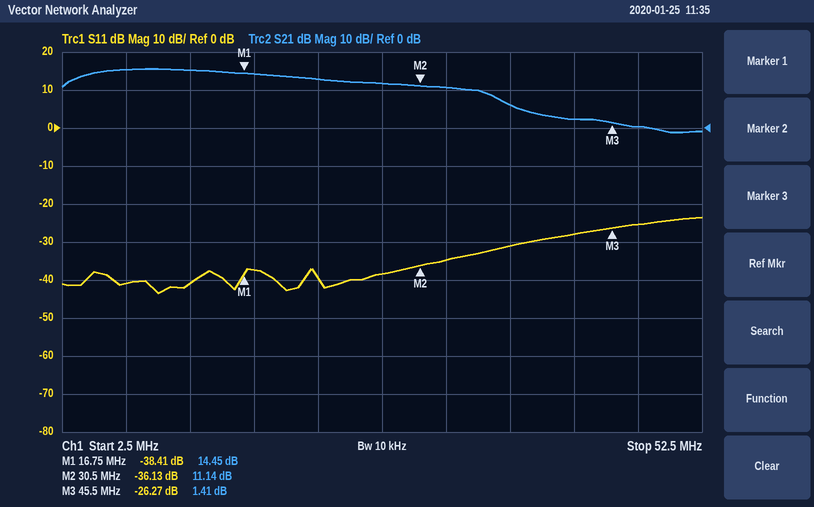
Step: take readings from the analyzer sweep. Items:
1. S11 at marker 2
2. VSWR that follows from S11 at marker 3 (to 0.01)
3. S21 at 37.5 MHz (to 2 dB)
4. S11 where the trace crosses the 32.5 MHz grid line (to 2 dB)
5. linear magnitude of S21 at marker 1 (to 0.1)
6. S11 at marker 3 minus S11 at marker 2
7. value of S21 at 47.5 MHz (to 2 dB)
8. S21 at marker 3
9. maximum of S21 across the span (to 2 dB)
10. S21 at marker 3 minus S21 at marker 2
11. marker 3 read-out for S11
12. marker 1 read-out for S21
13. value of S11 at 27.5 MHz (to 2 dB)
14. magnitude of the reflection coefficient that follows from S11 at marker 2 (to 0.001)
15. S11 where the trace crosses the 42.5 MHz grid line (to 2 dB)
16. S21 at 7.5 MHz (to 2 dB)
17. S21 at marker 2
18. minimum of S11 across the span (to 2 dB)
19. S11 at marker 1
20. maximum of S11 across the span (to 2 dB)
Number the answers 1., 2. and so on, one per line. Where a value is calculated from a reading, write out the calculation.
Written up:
1. -36.13 dB
2. (1 + 0.0486)/(1 − 0.0486) ≈ 1.10
3. 6 dB
4. -34 dB
5. 10^(14.45/20) ≈ 5.3
6. -26.27 − (-36.13) = 9.86 dB
7. 0 dB
8. 1.41 dB
9. 16 dB
10. 1.41 − (11.14) = -9.73 dB
11. -26.27 dB
12. 14.45 dB
13. -38 dB
14. 10^(-36.13/20) ≈ 0.016
15. -28 dB
16. 16 dB
17. 11.14 dB
18. -44 dB
19. -38.41 dB
20. -24 dB
